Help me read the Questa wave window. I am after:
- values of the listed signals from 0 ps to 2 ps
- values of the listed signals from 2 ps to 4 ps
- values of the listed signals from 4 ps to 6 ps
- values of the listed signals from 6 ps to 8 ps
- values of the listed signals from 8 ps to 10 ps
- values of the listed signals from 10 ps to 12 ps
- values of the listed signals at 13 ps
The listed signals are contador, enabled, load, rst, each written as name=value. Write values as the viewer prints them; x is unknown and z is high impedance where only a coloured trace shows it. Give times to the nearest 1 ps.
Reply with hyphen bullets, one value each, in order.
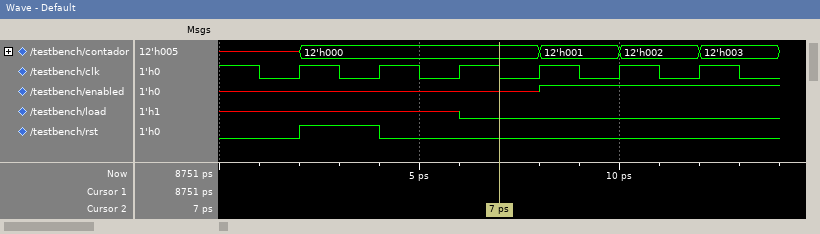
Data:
- contador=x, enabled=x, load=x, rst=0
- contador=12'h000, enabled=x, load=x, rst=1
- contador=12'h000, enabled=x, load=x, rst=0
- contador=12'h000, enabled=x, load=0, rst=0
- contador=12'h001, enabled=1, load=0, rst=0
- contador=12'h002, enabled=1, load=0, rst=0
- contador=12'h003, enabled=1, load=0, rst=0
